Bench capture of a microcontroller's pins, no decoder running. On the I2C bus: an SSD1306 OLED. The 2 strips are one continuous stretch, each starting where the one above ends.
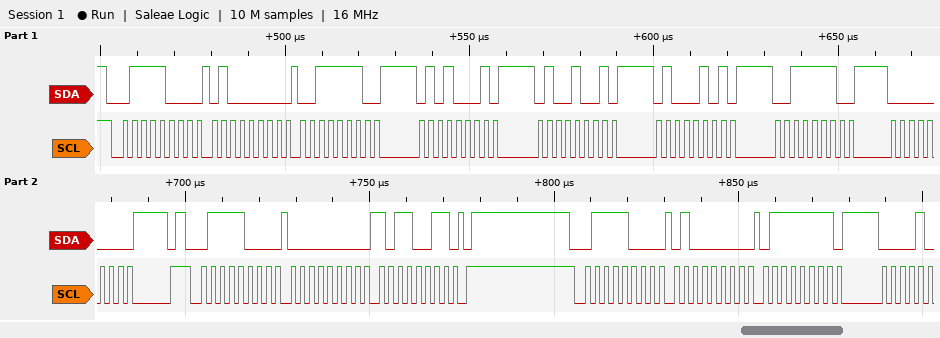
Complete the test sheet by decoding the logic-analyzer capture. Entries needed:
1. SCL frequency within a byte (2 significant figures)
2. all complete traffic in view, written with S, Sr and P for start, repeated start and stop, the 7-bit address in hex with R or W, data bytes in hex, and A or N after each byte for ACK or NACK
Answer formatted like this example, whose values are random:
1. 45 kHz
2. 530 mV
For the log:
1. 400 kHz
2. S 3CW A 40 A 3E A 51 A 49 A 45 A 3E A 00 A P S 3CW A 00 A B3 A P S 3CW A 40 A 7F A
